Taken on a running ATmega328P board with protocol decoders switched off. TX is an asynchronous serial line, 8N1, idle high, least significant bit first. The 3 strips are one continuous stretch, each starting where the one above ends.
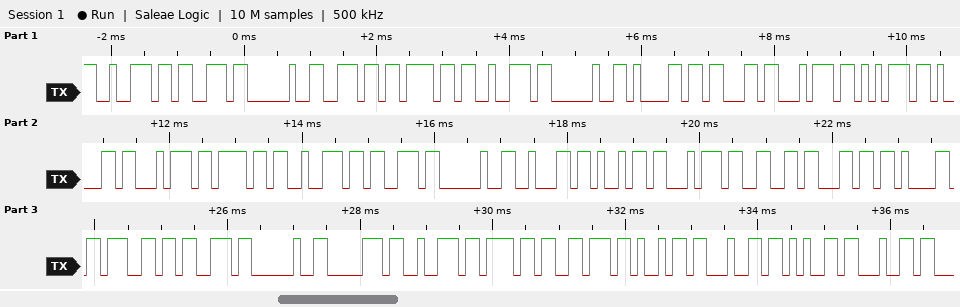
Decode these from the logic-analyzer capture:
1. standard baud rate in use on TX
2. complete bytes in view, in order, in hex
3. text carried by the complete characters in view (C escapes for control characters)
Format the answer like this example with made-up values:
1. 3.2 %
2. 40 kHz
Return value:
1. 9600 baud
2. 72 73 20 6E 6F 72 20 61 63 74 75 61 74 6F 72 73 20 62 69 74 66 6C 61 67 73 20 70 72 6F 76 69 64 65 64
3. "rs nor actuators bitflags provided"
